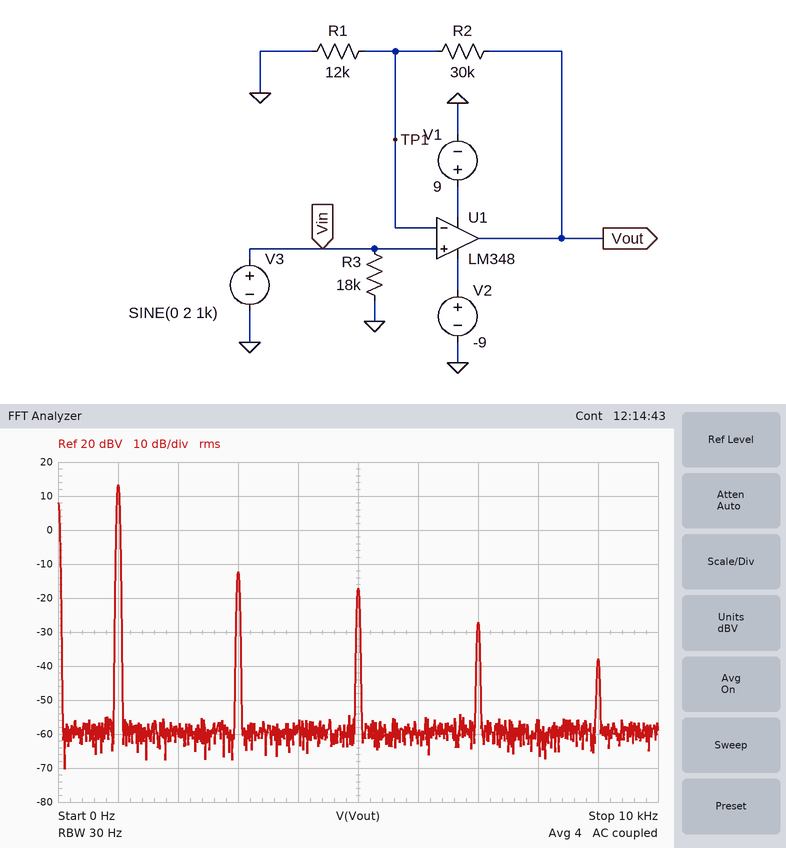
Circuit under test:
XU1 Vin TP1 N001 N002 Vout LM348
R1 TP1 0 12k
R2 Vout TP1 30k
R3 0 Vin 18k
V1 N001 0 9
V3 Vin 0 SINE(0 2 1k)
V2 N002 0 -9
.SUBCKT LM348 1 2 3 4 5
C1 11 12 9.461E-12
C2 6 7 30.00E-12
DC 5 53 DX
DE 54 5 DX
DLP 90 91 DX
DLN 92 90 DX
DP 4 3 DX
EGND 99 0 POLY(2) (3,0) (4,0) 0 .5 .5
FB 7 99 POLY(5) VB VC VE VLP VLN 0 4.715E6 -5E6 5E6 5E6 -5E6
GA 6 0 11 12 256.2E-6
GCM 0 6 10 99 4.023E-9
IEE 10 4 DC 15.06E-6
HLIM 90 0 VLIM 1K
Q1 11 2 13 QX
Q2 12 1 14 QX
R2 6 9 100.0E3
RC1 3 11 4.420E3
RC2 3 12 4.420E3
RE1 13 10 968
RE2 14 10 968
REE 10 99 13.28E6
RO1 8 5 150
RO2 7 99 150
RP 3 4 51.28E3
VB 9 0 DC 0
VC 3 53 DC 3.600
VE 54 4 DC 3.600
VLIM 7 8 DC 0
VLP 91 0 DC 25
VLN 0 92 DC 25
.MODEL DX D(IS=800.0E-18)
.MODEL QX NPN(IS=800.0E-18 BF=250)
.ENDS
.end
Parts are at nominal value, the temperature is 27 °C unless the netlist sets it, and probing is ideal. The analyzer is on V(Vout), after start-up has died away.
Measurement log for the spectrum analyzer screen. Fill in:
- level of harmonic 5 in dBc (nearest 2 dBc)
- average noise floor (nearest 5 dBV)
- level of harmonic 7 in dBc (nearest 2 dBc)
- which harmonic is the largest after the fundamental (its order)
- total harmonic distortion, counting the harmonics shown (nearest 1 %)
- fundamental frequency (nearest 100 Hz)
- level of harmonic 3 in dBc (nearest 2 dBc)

-30 dBc
-60 dBV
-40 dBc
3
6 %
1.0 kHz
-26 dBc
